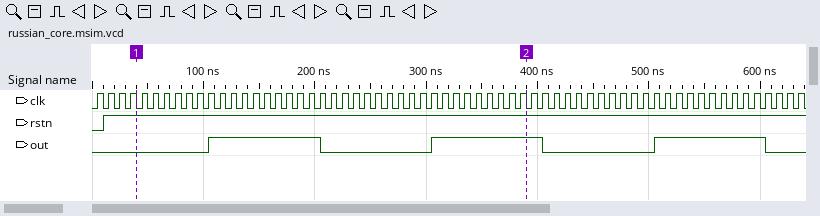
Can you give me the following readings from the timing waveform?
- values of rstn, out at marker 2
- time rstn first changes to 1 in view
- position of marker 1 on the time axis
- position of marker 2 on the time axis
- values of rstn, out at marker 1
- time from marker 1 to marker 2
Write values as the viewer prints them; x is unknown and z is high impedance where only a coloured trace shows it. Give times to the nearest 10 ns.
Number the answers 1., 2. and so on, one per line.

1. rstn=1, out=1
2. 10 ns
3. 40 ns
4. 390 ns
5. rstn=1, out=0
6. 350 ns
